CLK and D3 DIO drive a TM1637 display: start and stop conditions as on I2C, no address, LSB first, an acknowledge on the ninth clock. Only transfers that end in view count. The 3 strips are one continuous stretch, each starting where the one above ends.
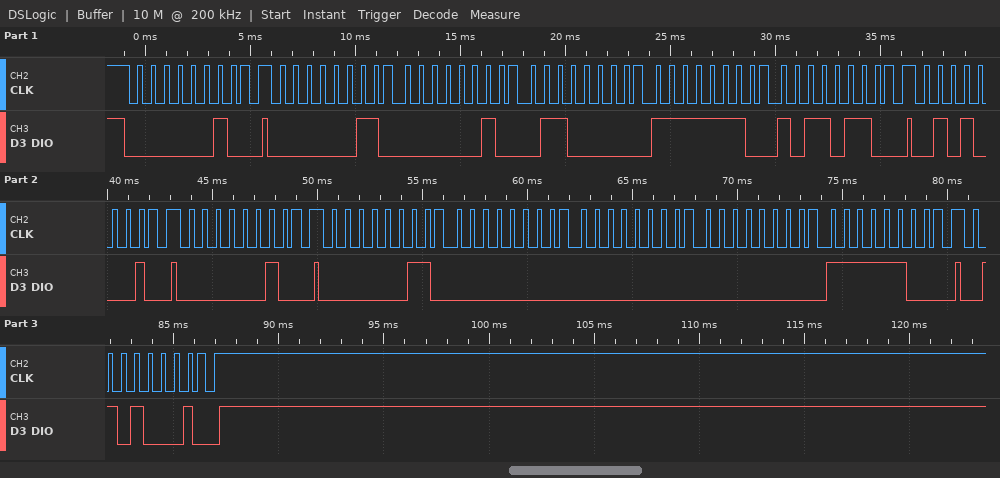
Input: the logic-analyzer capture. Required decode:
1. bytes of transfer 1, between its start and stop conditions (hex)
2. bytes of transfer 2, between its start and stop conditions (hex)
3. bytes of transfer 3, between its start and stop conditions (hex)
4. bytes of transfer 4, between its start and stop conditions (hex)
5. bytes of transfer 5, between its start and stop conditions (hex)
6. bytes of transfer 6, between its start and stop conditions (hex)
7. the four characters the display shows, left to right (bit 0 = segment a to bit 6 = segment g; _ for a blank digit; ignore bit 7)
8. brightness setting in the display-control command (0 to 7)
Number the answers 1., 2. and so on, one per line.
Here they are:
1. 40
2. C0 40 06 7F 6D
3. 8A
4. 40
5. C0 00 00 00 3F
6. 8A
7. ___0
8. 2
